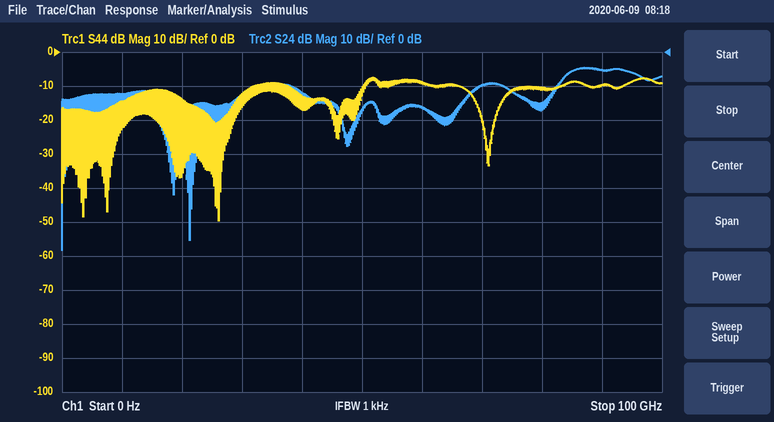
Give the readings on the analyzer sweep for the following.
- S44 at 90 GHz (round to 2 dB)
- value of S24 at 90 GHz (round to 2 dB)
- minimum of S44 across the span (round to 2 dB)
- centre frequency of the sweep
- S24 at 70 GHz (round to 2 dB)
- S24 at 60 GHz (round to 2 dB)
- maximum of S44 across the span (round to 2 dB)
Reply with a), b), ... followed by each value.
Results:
a) -10 dB
b) -6 dB
c) -50 dB
d) 50 GHz
e) -10 dB
f) -16 dB
g) -8 dB
